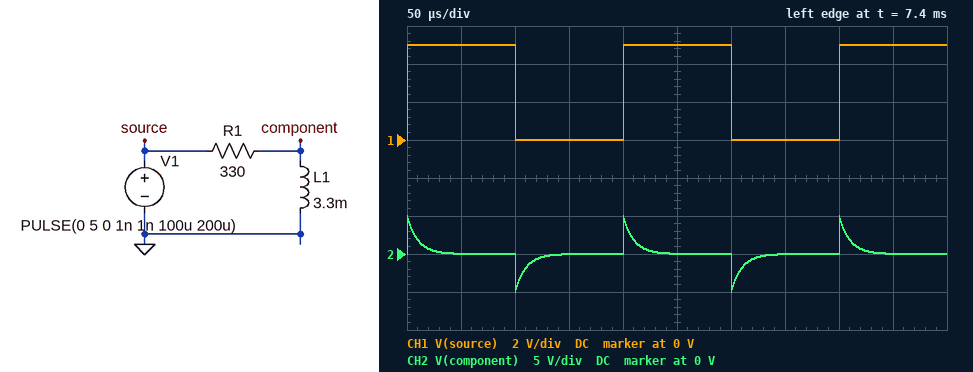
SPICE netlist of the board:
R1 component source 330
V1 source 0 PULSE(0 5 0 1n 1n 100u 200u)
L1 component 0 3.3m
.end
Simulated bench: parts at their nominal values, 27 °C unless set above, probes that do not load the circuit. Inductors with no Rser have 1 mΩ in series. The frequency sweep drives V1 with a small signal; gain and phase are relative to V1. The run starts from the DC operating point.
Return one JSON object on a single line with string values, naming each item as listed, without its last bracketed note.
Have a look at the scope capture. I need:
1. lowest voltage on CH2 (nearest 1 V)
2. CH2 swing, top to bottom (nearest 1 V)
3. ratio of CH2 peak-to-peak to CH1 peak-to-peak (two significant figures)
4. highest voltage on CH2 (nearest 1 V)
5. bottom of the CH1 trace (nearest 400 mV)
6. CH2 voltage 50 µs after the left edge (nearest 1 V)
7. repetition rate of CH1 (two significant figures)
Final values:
{"lowest voltage on CH2": "-5 V", "CH2 swing, top to bottom": "10 V", "ratio of CH2 peak-to-peak to CH1 peak-to-peak": "2.0", "highest voltage on CH2": "5 V", "bottom of the CH1 trace": "0 V", "CH2 voltage 50 µs after the left edge": "0 V", "repetition rate of CH1": "5.0 kHz"}
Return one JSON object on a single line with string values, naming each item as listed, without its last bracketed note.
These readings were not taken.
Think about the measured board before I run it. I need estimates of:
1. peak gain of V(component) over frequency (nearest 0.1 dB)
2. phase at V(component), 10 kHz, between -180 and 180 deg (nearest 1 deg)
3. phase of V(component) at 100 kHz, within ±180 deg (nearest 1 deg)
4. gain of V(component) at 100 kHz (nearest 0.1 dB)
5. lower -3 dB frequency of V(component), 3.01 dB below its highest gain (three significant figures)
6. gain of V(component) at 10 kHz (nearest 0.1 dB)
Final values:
{"peak gain of V(component) over frequency": "0 dB", "phase at V(component), 10 kHz, between -180 and 180 deg": "58 deg", "phase of V(component) at 100 kHz, within ±180 deg": "9 deg", "gain of V(component) at 100 kHz": "-0.1 dB", "lower -3 dB frequency of V(component), 3.01 dB below its highest gain": "15.9 kHz", "gain of V(component) at 10 kHz": "-5.5 dB"}
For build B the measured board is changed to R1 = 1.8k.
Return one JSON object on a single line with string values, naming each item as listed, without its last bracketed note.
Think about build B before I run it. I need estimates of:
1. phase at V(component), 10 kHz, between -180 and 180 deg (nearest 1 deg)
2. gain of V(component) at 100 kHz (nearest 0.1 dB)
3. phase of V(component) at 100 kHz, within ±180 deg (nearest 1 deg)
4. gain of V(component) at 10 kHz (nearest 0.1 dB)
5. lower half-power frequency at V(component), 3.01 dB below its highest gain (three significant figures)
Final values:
{"phase at V(component), 10 kHz, between -180 and 180 deg": "83 deg", "gain of V(component) at 100 kHz": "-2.4 dB", "phase of V(component) at 100 kHz, within ±180 deg": "41 deg", "gain of V(component) at 10 kHz": "-18.8 dB", "lower half-power frequency at V(component), 3.01 dB below its highest gain": "86.8 kHz"}
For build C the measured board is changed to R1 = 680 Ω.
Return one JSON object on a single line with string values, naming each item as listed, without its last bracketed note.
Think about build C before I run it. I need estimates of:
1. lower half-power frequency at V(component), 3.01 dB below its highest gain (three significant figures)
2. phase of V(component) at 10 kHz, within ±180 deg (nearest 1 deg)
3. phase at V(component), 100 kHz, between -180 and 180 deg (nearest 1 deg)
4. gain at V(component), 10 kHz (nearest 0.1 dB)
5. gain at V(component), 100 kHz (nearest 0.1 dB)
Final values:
{"lower half-power frequency at V(component), 3.01 dB below its highest gain": "32.8 kHz", "phase of V(component) at 10 kHz, within ±180 deg": "73 deg", "phase at V(component), 100 kHz, between -180 and 180 deg": "18 deg", "gain at V(component), 10 kHz": "-10.7 dB", "gain at V(component), 100 kHz": "-0.4 dB"}
